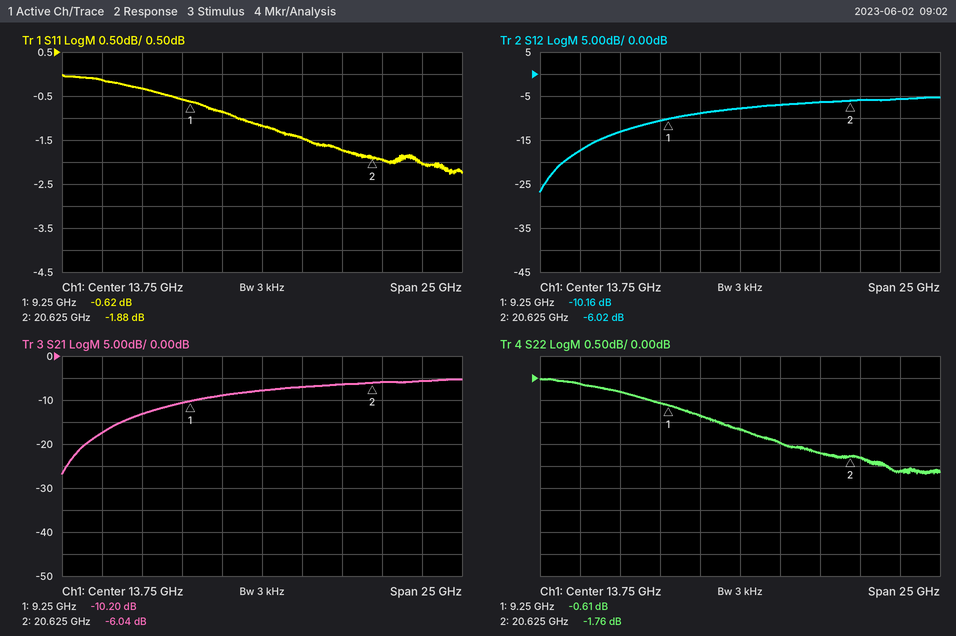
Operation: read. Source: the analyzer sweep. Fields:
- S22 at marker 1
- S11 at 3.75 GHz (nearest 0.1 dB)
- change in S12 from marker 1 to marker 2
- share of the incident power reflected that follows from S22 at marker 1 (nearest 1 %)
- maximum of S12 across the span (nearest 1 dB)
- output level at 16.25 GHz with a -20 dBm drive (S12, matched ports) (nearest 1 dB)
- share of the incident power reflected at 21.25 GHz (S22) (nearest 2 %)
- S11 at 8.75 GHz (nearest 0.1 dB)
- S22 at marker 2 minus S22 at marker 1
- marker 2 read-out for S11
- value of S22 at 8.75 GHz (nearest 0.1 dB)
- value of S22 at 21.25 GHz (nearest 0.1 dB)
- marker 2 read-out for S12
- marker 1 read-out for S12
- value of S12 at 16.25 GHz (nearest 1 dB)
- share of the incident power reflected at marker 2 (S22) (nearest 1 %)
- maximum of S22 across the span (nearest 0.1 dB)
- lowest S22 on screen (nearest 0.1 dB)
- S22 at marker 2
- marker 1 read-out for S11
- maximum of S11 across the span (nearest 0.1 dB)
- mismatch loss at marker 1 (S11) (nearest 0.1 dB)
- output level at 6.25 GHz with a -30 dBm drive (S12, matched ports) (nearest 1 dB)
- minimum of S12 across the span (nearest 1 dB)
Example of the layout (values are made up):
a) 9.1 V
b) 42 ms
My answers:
a) -0.61 dB
b) -0.1 dB
c) 4.14 dB
d) 87 %
e) -5 dB
f) -27 dBm
g) 66 %
h) -0.6 dB
i) -1.15 dB
j) -1.88 dB
k) -0.6 dB
l) -1.8 dB
m) -6.02 dB
n) -10.16 dB
o) -7 dB
p) 67 %
q) 0.0 dB
r) -2.2 dB
s) -1.76 dB
t) -0.62 dB
u) 0.0 dB
v) 8.8 dB
w) -43 dBm
x) -27 dB
